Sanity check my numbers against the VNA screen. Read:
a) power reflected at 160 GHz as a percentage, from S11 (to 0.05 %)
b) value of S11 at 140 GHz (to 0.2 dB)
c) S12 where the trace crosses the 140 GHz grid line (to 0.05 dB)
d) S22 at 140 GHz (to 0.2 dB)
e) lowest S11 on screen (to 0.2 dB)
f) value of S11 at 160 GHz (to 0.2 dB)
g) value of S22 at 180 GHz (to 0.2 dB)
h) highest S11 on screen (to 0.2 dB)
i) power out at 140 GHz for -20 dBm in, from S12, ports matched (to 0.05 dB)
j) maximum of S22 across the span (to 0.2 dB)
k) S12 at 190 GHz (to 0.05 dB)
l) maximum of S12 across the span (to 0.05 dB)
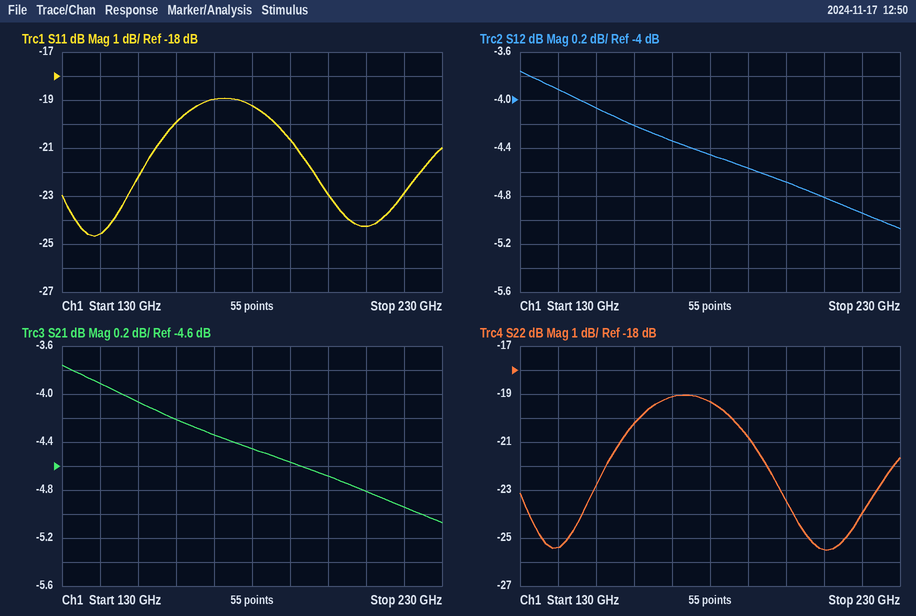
1.00 %
-24.6 dB
-3.90 dB
-25.4 dB
-24.6 dB
-20.0 dB
-19.4 dB
-19.0 dB
-23.90 dBm
-19.0 dB
-4.55 dB
-3.75 dB
